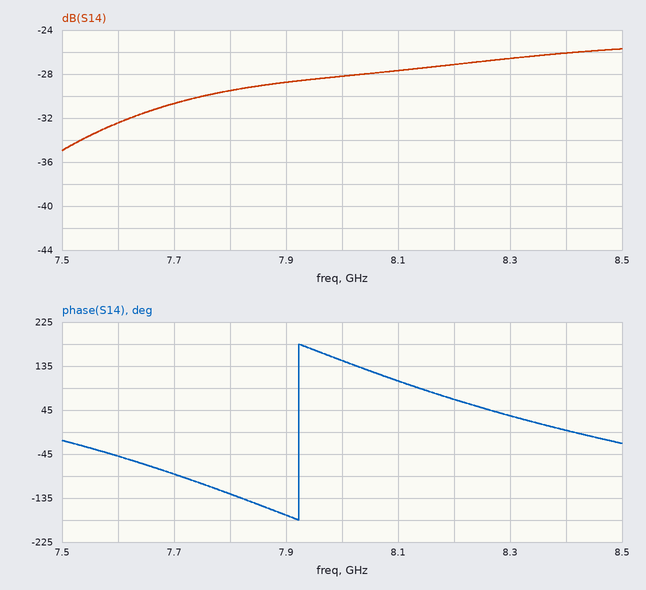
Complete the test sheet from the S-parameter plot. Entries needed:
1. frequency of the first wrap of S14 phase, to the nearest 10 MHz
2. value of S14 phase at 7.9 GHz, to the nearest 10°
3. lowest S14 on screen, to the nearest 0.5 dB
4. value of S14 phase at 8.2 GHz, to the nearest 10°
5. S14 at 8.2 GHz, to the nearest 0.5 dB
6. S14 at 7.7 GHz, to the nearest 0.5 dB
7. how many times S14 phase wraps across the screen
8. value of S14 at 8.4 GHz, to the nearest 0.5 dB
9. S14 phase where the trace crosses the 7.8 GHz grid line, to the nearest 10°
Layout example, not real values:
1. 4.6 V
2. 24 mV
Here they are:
1. 7.92 GHz
2. -170°
3. -35.0 dB
4. 70°
5. -27.0 dB
6. -30.5 dB
7. 1
8. -26.0 dB
9. -130°
